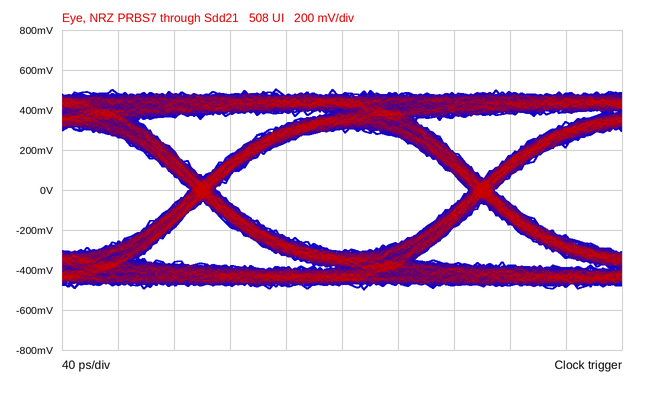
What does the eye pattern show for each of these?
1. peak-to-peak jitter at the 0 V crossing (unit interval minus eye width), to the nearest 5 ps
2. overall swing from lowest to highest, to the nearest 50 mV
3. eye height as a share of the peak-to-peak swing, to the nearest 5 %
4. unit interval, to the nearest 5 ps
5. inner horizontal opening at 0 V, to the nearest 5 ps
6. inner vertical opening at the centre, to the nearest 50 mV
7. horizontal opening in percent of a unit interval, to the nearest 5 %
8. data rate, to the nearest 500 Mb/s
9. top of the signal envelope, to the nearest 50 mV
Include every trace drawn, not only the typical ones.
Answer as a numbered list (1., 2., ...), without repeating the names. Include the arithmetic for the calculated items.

1. 20 ps
2. 1.00 V
3. 600 mV / 1.00 V ≈ 60 %
4. 200 ps
5. 180 ps
6. 600 mV
7. 180 ps / 200 ps ≈ 90 %
8. 5.0 Gb/s
9. 500 mV
